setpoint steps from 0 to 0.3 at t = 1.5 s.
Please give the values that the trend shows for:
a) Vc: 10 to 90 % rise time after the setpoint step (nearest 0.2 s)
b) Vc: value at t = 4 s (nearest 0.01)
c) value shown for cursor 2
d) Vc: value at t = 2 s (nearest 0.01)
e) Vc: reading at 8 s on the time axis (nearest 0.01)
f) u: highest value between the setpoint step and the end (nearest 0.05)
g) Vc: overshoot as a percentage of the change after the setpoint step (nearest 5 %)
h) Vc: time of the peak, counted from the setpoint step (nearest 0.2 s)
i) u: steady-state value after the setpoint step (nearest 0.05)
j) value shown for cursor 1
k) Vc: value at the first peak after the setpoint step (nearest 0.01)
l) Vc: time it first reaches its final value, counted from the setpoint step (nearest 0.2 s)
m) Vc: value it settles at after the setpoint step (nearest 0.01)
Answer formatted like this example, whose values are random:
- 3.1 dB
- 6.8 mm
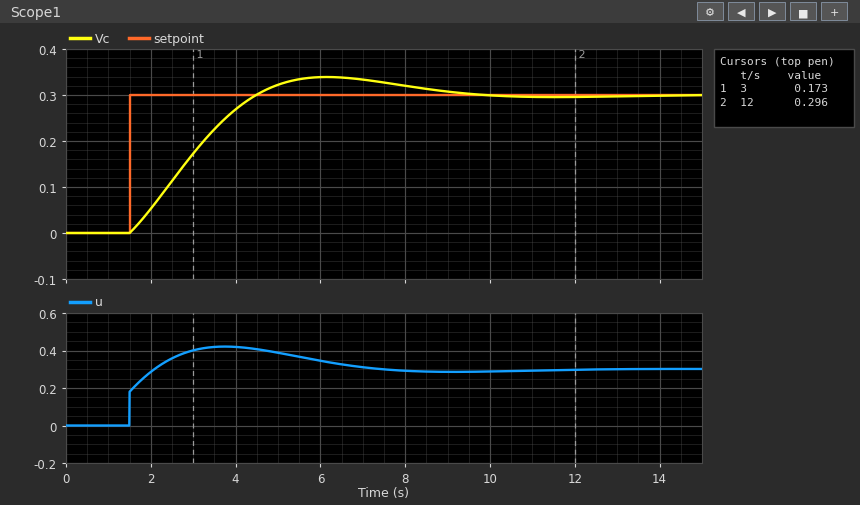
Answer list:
- 2.2 s
- 0.27
- 0.296
- 0.05
- 0.32
- 0.40
- 15 %
- 4.6 s
- 0.30
- 0.173
- 0.34
- 3.0 s
- 0.30
